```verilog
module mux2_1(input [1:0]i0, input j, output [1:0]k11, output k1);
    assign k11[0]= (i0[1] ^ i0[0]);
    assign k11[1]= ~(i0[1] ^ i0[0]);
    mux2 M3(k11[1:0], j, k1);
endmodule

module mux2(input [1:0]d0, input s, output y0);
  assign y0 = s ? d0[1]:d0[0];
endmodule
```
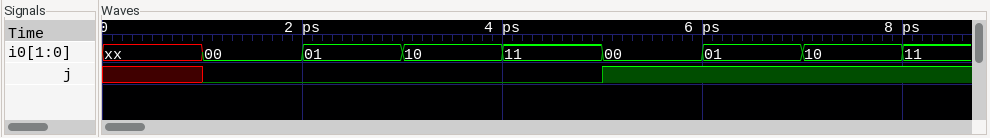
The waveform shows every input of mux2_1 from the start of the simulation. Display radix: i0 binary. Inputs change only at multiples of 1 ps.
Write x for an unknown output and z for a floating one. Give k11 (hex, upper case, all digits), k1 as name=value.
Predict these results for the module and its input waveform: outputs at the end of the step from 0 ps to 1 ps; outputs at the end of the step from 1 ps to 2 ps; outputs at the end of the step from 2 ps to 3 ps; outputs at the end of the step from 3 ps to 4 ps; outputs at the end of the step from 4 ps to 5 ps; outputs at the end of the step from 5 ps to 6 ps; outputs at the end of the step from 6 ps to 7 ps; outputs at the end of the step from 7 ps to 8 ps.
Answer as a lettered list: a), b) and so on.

a) k11=x, k1=x
b) k11=2, k1=0
c) k11=1, k1=1
d) k11=1, k1=1
e) k11=2, k1=0
f) k11=2, k1=1
g) k11=1, k1=0
h) k11=1, k1=0
